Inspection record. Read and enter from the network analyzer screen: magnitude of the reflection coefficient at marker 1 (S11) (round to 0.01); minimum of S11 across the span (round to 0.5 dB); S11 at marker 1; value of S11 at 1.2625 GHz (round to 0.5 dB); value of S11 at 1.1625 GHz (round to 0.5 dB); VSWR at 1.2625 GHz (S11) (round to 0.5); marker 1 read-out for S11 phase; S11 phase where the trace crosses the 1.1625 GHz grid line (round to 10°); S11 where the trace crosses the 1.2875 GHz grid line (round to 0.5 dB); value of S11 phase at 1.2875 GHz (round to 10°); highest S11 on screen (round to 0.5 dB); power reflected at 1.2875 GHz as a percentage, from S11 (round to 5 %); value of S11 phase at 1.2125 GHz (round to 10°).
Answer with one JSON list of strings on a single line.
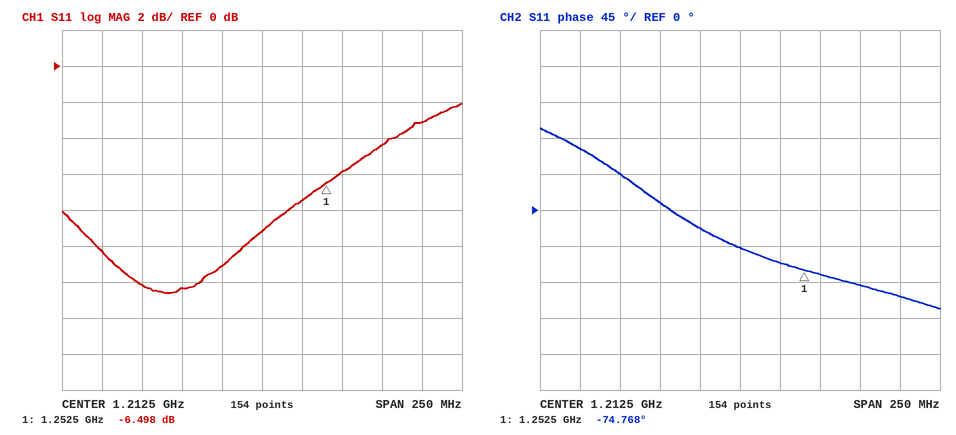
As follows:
["0.47", "-12.5 dB", "-6.498 dB", "-6.0 dB", "-12.5 dB", "3.0", "-74.768°", "10°", "-4.5 dB", "-90°", "-2.0 dB", "35 %", "-50°"]
